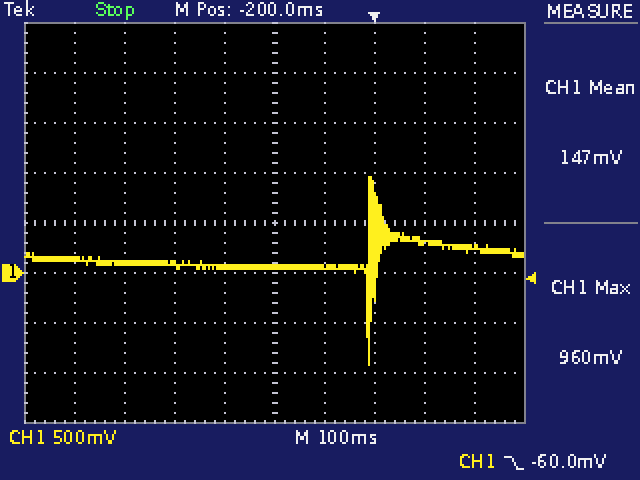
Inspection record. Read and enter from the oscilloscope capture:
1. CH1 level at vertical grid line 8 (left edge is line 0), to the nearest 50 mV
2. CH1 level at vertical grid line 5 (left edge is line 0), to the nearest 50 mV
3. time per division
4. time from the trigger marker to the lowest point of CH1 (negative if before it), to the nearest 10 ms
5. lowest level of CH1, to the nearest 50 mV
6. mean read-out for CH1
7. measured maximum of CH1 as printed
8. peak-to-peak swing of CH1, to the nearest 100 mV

300 mV
50 mV
100 ms
-10 ms
-900 mV
147 mV
960 mV
1.90 V
